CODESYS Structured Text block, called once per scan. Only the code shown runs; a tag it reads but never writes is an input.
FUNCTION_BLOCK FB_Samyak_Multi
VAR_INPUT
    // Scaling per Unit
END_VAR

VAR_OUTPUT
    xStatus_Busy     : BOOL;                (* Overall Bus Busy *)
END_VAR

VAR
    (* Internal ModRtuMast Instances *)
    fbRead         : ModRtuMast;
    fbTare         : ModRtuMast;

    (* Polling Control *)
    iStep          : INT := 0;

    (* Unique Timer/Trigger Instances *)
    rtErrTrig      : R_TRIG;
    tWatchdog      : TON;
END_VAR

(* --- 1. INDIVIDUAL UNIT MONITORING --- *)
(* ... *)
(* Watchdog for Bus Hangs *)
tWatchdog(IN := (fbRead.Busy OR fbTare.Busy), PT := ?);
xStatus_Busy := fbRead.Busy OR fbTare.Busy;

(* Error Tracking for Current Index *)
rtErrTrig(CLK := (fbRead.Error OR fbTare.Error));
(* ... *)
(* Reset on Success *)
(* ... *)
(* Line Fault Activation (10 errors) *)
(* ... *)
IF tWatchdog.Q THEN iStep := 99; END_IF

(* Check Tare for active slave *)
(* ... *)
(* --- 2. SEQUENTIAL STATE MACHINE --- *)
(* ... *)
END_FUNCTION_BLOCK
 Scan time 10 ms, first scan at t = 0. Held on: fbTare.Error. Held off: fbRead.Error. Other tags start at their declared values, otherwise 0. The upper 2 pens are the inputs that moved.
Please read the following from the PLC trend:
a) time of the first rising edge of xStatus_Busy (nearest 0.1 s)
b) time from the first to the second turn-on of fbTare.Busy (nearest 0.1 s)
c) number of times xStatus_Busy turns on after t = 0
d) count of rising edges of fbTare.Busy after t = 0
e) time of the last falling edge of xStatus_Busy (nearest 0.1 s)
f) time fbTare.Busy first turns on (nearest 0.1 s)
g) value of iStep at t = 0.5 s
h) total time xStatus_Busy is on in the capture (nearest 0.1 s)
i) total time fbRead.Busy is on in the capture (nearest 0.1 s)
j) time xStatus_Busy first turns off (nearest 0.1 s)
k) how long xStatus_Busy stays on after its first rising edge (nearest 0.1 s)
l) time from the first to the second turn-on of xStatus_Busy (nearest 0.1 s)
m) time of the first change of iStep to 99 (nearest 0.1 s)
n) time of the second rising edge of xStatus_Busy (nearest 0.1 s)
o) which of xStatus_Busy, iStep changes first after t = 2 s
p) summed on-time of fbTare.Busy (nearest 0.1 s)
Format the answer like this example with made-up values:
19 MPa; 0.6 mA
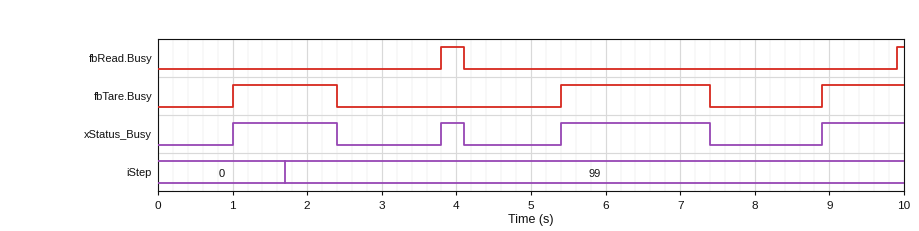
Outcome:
1.0 s; 4.4 s; 4; 3; 7.4 s; 1.0 s; 0; 4.8 s; 0.4 s; 2.4 s; 1.4 s; 2.8 s; 1.7 s; 3.8 s; xStatus_Busy; 4.5 s
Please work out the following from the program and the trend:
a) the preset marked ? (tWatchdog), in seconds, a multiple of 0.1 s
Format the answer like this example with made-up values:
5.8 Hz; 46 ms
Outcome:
0.7 s
